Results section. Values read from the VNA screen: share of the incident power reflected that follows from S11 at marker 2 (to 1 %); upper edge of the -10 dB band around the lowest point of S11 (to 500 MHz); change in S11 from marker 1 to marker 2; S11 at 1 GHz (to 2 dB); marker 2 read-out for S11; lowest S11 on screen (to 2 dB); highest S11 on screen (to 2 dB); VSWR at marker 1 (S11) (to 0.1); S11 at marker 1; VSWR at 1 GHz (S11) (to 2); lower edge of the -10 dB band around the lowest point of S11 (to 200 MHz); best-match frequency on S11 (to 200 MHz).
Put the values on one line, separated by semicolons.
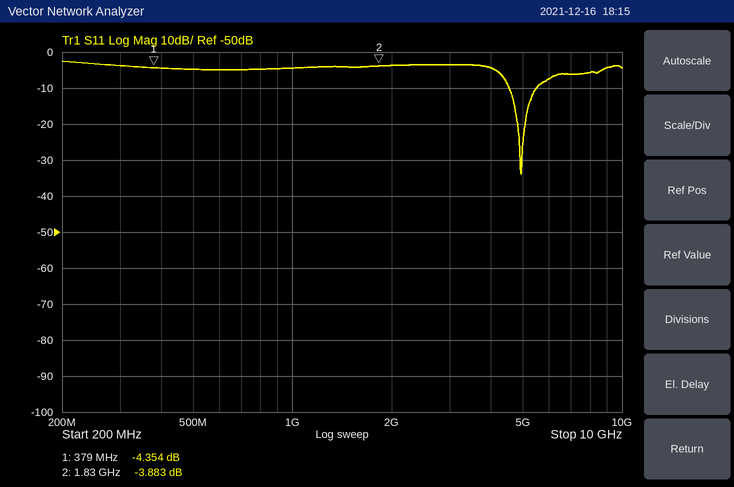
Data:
41 %; 5.5 GHz; 0.471 dB; -4 dB; -3.883 dB; -34 dB; -2 dB; 4.1; -4.354 dB; 4; 4.6 GHz; 5.0 GHz
